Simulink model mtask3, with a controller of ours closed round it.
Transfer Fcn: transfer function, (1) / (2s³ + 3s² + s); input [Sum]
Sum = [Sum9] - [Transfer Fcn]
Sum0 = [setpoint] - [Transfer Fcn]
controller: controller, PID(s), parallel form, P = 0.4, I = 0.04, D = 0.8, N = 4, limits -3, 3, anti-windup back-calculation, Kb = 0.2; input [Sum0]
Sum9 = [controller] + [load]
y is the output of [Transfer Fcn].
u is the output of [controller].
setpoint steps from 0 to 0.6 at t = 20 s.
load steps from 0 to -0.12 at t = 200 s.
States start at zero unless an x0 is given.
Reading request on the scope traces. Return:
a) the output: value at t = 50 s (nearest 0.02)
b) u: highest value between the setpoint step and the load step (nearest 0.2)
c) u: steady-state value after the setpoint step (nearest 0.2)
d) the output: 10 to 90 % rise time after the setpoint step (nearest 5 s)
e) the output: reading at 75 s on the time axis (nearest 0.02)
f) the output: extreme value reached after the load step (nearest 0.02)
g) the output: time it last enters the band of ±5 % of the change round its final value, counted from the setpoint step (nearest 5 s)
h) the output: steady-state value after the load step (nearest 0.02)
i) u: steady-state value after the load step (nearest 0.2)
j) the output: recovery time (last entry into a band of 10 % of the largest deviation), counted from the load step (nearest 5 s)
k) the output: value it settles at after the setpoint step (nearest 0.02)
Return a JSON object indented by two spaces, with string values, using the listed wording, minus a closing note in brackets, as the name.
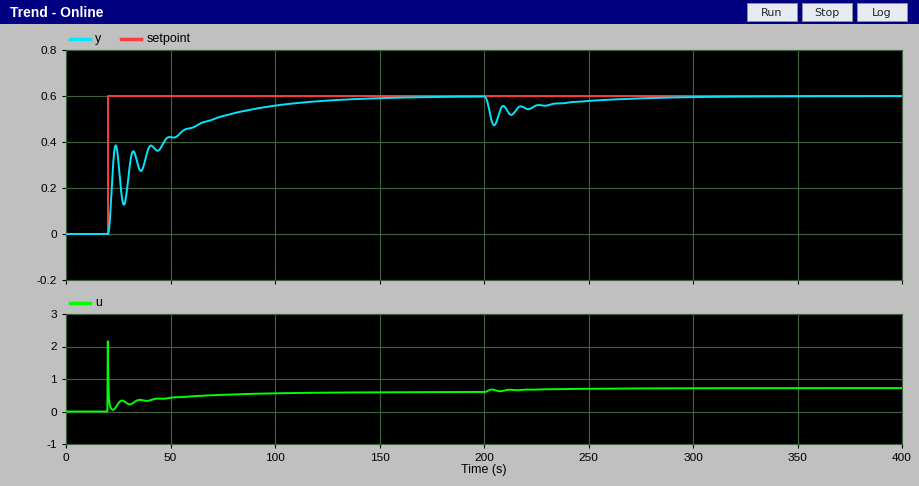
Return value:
{
  "the output: value at t = 50 s": "0.42",
  "u: highest value between the setpoint step and the load step": "2.2",
  "u: steady-state value after the setpoint step": "0.6",
  "the output: 10 to 90 % rise time after the setpoint step": "65 s",
  "the output: reading at 75 s on the time axis": "0.52",
  "the output: extreme value reached after the load step": "0.48",
  "the output: time it last enters the band of ±5 % of the change round its final value, counted from the setpoint step": "90 s",
  "the output: steady-state value after the load step": "0.60",
  "u: steady-state value after the load step": "0.8",
  "the output: recovery time (last entry into a band of 10 % of the largest deviation), counted from the load step": "70 s",
  "the output: value it settles at after the setpoint step": "0.60"
}
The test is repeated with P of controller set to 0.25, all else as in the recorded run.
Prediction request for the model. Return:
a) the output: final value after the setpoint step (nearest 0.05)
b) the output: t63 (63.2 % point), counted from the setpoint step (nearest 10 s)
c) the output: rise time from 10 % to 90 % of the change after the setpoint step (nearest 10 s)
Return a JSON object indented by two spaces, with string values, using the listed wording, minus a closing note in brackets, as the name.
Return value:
{
  "the output: final value after the setpoint step": "0.60",
  "the output: t63 (63.2 % point), counted from the setpoint step": "30 s",
  "the output: rise time from 10 % to 90 % of the change after the setpoint step": "60 s"
}
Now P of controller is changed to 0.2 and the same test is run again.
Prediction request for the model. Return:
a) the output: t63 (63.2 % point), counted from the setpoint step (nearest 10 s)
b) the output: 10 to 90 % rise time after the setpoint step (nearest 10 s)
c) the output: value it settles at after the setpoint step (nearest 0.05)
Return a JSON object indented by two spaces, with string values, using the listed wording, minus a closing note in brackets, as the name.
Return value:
{
  "the output: t63 (63.2 % point), counted from the setpoint step": "30 s",
  "the output: 10 to 90 % rise time after the setpoint step": "60 s",
  "the output: value it settles at after the setpoint step": "0.60"
}
